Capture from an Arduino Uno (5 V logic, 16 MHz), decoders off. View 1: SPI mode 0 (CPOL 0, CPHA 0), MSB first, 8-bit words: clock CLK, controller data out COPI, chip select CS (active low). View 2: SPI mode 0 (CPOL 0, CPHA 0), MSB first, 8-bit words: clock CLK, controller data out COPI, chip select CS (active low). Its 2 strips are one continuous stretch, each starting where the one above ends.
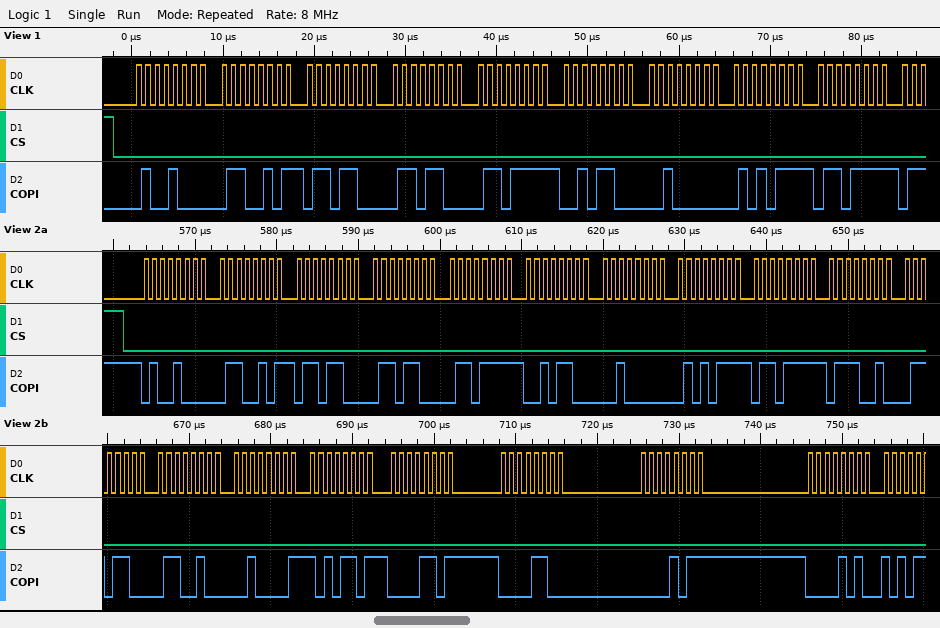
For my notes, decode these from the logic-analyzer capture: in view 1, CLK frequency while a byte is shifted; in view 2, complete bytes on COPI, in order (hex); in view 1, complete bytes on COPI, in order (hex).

1 MHz
48 65 6C 6C 6F 2C 20 57 6F 72 6C 64 21 AD 0D 0C 0B 0A
48 65 6C 6C 6F 2C 20 57 6F
